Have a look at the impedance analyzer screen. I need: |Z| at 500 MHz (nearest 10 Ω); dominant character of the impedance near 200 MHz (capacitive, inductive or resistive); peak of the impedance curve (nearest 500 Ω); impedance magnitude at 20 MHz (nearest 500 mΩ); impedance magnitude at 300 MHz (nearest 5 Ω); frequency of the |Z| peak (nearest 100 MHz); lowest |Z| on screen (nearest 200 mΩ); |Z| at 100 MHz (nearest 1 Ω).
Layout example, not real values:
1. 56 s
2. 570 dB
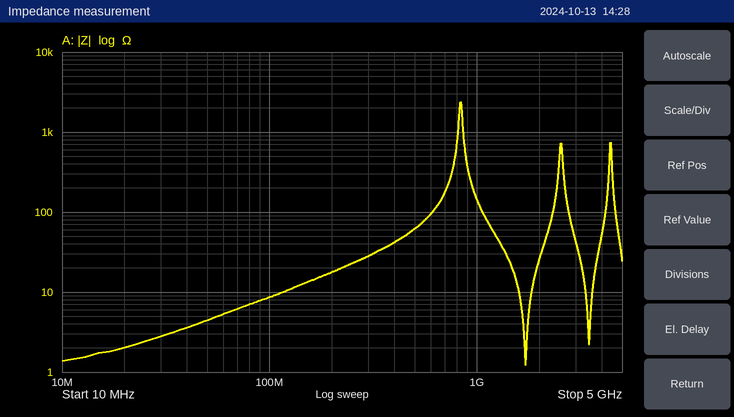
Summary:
1. 60 Ω
2. inductive
3. 2.5 kΩ
4. 2.0 Ω
5. 30 Ω
6. 800 MHz
7. 1.2 Ω
8. 9 Ω
